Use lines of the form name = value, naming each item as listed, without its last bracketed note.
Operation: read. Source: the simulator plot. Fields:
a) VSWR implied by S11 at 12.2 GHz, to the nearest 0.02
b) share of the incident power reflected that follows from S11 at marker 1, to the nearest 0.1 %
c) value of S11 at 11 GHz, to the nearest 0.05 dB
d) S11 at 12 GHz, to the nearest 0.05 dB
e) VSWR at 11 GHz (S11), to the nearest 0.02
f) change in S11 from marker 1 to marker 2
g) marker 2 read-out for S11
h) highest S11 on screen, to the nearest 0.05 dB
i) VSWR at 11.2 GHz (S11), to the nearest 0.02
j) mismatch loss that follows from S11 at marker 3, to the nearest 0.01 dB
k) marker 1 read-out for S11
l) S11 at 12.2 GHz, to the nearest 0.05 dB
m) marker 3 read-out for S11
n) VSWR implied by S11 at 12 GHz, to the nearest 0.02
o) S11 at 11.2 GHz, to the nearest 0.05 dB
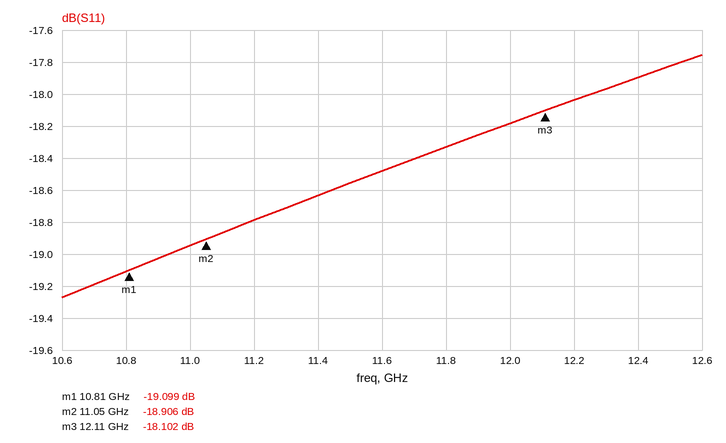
VSWR implied by S11 at 12.2 GHz, to the nearest 0.02 = 1.28
share of the incident power reflected that follows from S11 at marker 1, to the nearest 0.1 % = 1.2 %
value of S11 at 11 GHz, to the nearest 0.05 dB = -18.95 dB
S11 at 12 GHz, to the nearest 0.05 dB = -18.20 dB
VSWR at 11 GHz (S11), to the nearest 0.02 = 1.26
change in S11 from marker 1 to marker 2 = 0.193 dB
marker 2 read-out for S11 = -18.906 dB
highest S11 on screen, to the nearest 0.05 dB = -17.75 dB
VSWR at 11.2 GHz (S11), to the nearest 0.02 = 1.26
mismatch loss that follows from S11 at marker 3, to the nearest 0.01 dB = 0.07 dB
marker 1 read-out for S11 = -19.099 dB
S11 at 12.2 GHz, to the nearest 0.05 dB = -18.05 dB
marker 3 read-out for S11 = -18.102 dB
VSWR implied by S11 at 12 GHz, to the nearest 0.02 = 1.28
S11 at 11.2 GHz, to the nearest 0.05 dB = -18.80 dB
